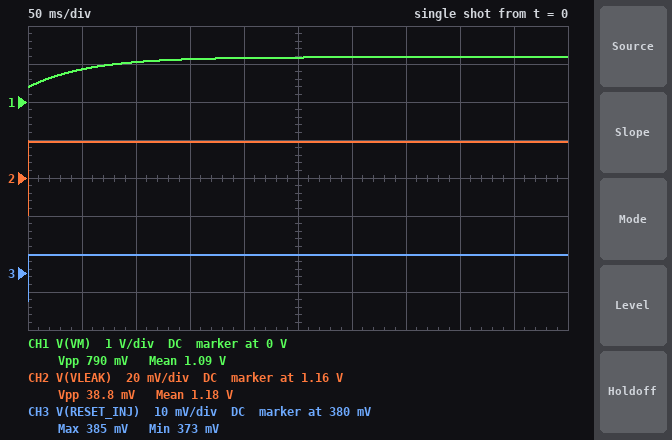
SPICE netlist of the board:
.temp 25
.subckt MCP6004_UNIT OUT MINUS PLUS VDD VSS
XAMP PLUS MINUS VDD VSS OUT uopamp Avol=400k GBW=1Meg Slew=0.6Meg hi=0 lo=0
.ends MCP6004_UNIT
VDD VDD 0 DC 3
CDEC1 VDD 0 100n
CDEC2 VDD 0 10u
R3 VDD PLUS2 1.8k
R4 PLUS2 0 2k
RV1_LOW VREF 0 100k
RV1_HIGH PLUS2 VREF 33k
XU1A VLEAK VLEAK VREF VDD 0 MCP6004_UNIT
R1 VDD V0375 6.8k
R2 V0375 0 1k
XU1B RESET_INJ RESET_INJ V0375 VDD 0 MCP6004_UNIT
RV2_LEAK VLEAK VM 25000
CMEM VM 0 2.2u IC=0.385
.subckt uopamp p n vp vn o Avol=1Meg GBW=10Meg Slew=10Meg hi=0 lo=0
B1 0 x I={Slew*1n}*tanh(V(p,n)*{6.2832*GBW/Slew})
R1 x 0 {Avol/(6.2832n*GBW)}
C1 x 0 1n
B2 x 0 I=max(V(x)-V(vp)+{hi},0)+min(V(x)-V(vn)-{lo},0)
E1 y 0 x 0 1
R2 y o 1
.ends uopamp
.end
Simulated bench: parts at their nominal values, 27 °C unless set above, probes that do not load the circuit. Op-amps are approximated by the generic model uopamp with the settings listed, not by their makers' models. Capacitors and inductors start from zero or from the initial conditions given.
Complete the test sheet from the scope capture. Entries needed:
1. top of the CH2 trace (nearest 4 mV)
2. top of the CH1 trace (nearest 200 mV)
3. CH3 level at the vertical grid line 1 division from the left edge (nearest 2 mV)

1.180 V
1.2 V
384 mV
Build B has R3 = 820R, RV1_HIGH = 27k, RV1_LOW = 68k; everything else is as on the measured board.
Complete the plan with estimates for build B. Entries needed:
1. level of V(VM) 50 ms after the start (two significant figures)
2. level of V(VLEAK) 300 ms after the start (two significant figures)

1.1 V
1.5 V
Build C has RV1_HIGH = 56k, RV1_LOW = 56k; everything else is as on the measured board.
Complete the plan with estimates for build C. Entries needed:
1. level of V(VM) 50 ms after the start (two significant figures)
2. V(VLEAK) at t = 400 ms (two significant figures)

620 mV
780 mV
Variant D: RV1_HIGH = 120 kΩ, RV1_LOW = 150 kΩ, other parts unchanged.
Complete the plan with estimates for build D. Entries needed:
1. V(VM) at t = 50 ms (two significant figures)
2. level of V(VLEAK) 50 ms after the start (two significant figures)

680 mV
870 mV
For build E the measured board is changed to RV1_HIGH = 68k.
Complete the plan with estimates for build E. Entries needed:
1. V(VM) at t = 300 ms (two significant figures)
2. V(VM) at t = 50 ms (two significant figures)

930 mV
710 mV
